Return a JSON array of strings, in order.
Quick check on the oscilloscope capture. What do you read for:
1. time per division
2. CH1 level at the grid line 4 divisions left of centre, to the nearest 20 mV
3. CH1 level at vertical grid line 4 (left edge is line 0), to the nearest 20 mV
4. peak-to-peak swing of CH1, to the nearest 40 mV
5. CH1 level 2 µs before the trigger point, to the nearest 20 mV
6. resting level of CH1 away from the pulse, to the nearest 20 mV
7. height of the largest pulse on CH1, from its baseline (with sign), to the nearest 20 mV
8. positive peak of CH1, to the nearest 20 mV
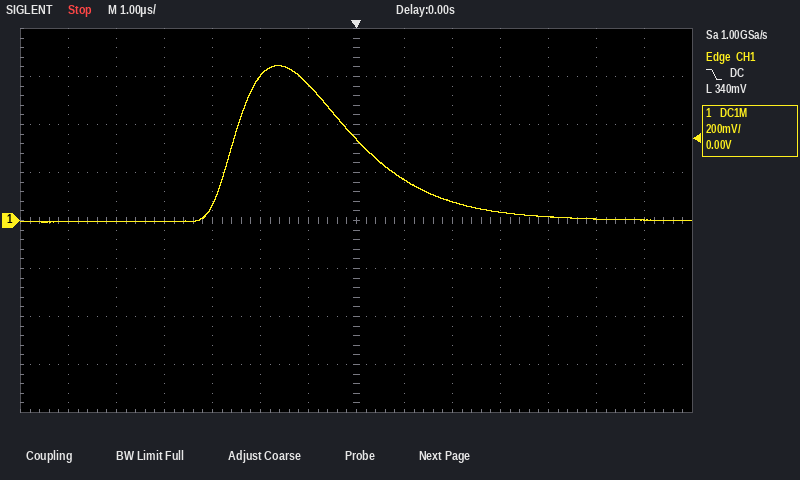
["1 µs", "0 mV", "60 mV", "640 mV", "600 mV", "0 mV", "+640 mV", "640 mV"]
